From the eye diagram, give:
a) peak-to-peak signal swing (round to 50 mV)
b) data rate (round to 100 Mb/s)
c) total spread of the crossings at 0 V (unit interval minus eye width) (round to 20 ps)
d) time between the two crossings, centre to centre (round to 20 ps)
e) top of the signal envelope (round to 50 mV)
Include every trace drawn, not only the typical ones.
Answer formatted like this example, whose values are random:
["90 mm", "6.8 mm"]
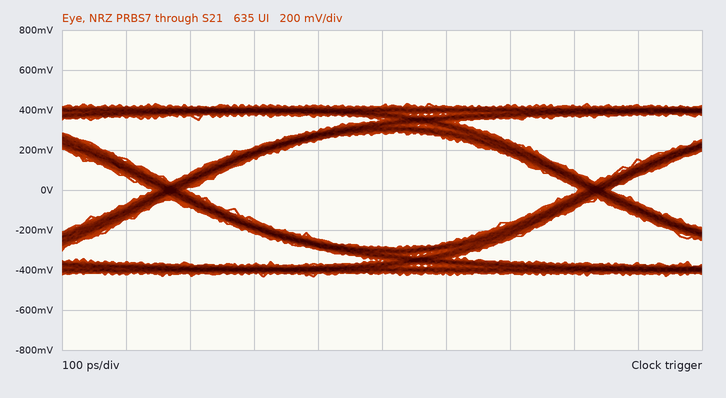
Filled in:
["850 mV", "1.5 Gb/s", "60 ps", "660 ps", "450 mV"]
